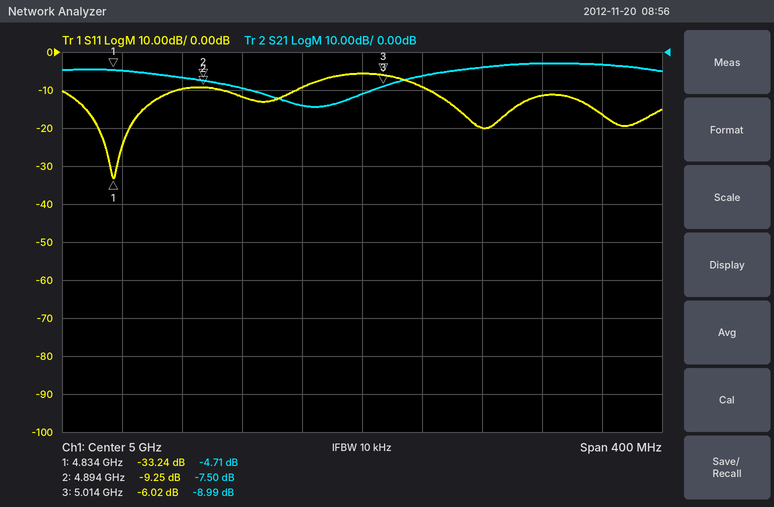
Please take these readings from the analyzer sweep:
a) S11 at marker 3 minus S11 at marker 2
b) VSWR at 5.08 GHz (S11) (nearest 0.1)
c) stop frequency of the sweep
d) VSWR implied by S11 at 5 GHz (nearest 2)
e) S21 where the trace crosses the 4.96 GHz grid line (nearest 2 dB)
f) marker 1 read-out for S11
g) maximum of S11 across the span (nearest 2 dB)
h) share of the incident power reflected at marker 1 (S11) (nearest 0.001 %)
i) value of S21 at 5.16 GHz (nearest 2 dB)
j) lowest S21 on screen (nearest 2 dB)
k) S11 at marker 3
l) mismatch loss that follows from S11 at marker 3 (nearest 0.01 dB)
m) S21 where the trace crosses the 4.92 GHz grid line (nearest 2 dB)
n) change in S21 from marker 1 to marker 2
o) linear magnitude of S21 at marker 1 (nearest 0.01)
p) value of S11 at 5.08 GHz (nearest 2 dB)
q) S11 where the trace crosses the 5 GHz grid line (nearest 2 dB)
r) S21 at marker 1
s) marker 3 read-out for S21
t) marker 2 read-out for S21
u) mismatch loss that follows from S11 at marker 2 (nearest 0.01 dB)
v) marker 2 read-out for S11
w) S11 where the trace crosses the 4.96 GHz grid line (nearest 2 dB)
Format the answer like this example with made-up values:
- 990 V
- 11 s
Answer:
- 3.23 dB
- 1.2
- 5.2 GHz
- 4
- -14 dB
- -33.24 dB
- -6 dB
- 0.047 %
- -4 dB
- -14 dB
- -6.02 dB
- 1.25 dB
- -10 dB
- -2.79 dB
- 0.58
- -20 dB
- -6 dB
- -4.71 dB
- -8.99 dB
- -7.50 dB
- 0.55 dB
- -9.25 dB
- -10 dB
